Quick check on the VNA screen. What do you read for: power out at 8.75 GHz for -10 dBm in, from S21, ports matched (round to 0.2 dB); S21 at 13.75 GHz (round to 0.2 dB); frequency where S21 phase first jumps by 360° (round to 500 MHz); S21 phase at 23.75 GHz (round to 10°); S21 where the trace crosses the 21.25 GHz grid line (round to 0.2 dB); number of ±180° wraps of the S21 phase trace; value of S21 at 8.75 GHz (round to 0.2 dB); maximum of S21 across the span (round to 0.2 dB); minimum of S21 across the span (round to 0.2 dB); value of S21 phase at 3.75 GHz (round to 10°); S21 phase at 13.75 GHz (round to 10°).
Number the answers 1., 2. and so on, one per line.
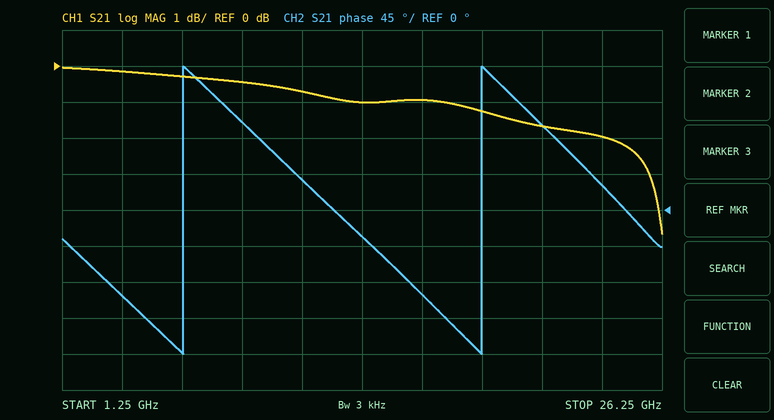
1. -10.4 dBm
2. -1.0 dB
3. 6.5 GHz
4. 30°
5. -1.6 dB
6. 2
7. -0.4 dB
8. 0.0 dB
9. -4.6 dB
10. -110°
11. -30°
